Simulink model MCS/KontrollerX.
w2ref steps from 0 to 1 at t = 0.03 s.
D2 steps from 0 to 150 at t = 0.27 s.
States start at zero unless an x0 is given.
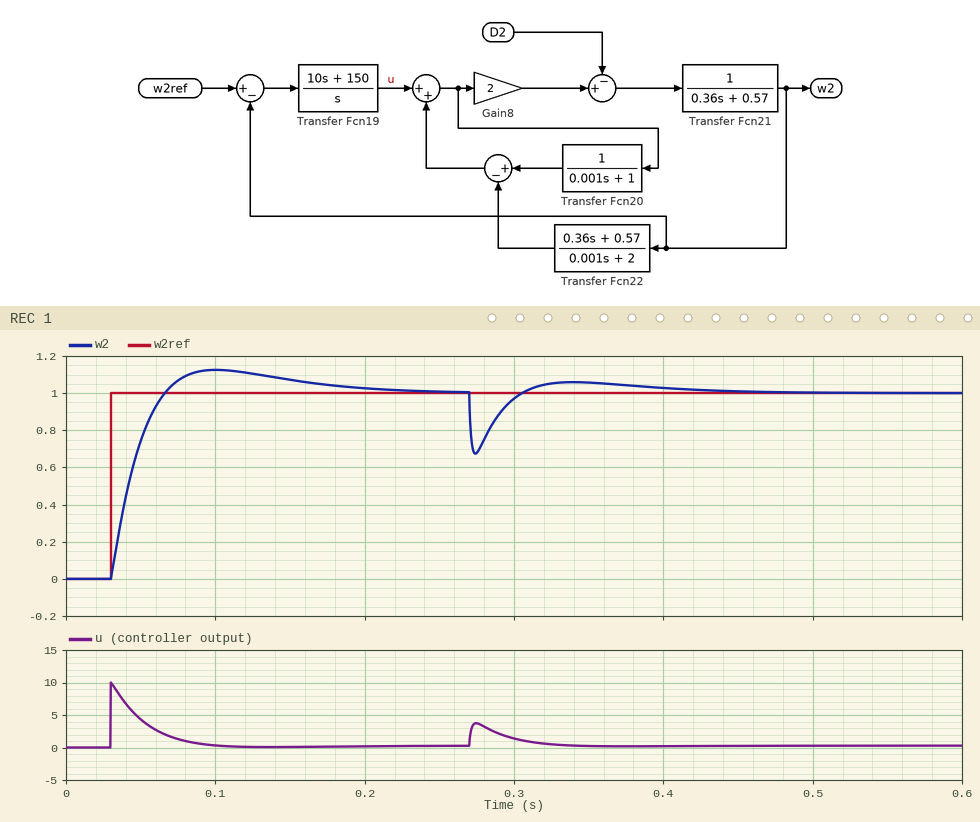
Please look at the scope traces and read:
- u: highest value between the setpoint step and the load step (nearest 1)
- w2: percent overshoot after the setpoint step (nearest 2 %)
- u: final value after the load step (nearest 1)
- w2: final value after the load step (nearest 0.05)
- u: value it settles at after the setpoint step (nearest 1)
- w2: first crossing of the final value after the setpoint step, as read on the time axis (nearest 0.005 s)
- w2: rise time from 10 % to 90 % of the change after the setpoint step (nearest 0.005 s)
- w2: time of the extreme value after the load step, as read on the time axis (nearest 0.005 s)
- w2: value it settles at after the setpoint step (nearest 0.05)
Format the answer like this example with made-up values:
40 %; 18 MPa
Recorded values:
10; 12 %; 0; 1.00; 0; 0.065 s; 0.025 s; 0.275 s; 1.00
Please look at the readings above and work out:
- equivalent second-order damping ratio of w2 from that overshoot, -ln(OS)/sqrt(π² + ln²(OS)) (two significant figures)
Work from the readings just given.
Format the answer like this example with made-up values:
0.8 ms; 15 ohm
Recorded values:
0.56
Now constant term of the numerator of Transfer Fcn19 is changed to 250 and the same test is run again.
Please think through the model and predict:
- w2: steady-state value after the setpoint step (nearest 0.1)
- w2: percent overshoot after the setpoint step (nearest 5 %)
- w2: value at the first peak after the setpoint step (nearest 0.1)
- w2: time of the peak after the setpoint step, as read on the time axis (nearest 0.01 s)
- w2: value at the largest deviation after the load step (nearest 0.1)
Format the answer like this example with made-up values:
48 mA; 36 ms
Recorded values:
1.0; 20 %; 1.2; 0.09 s; 0.7
